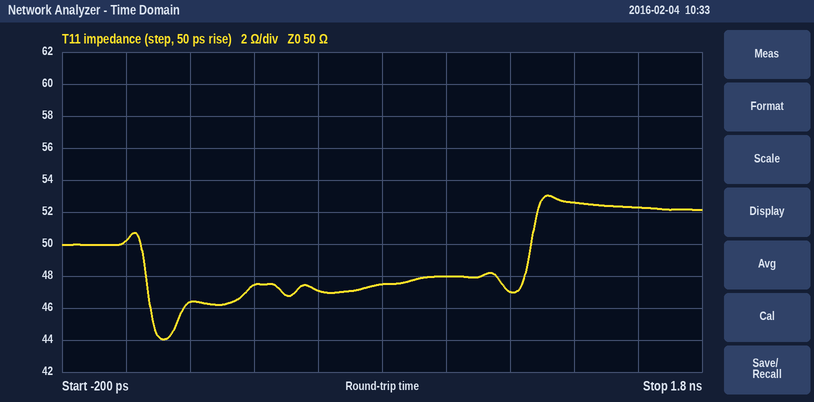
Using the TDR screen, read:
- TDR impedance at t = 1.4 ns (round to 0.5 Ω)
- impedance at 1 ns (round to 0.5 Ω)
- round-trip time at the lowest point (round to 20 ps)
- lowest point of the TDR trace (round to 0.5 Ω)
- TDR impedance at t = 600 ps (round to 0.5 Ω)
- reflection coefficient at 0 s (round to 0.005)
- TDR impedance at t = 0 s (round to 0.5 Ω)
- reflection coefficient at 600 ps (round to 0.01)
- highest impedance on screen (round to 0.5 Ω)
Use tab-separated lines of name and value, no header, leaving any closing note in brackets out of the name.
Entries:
TDR impedance at t = 1.4 ns	52.5 Ω
impedance at 1 ns	48.0 Ω
round-trip time at the lowest point	120 ps
lowest point of the TDR trace	44.0 Ω
TDR impedance at t = 600 ps	47.0 Ω
reflection coefficient at 0 s	0.000
TDR impedance at t = 0 s	50.0 Ω
reflection coefficient at 600 ps	-0.03
highest impedance on screen	53.0 Ω
